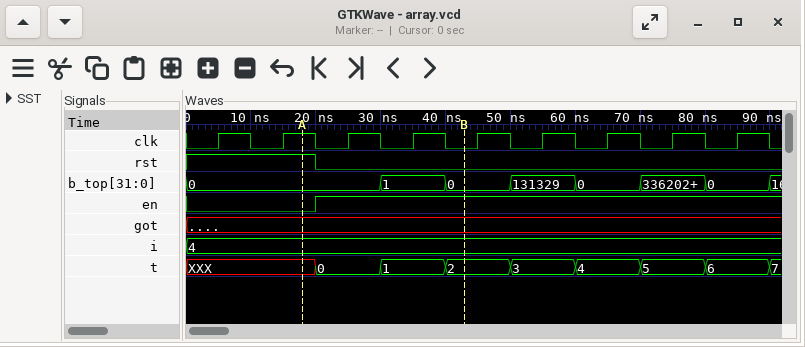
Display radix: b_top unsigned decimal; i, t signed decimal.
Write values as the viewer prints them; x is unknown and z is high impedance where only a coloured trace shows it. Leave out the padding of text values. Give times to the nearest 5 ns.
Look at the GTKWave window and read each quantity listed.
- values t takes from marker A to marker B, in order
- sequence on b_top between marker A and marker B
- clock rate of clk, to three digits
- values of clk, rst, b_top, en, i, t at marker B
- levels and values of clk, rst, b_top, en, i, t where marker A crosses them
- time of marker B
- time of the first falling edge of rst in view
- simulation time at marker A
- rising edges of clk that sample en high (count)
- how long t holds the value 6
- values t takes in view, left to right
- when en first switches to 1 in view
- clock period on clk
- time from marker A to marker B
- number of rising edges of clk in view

XXX, 0, 1, 2
0, 1, 0
100 MHz
clk=0, rst=0, b_top=0, en=1, i=4, t=2
clk=1, rst=1, b_top=0, en=0, i=4, t=XXX
45 ns
20 ns
20 ns
7
10 ns
XXX, 0, 1, 2, 3, 4, 5, 6, 7
20 ns
10 ns
25 ns
9
